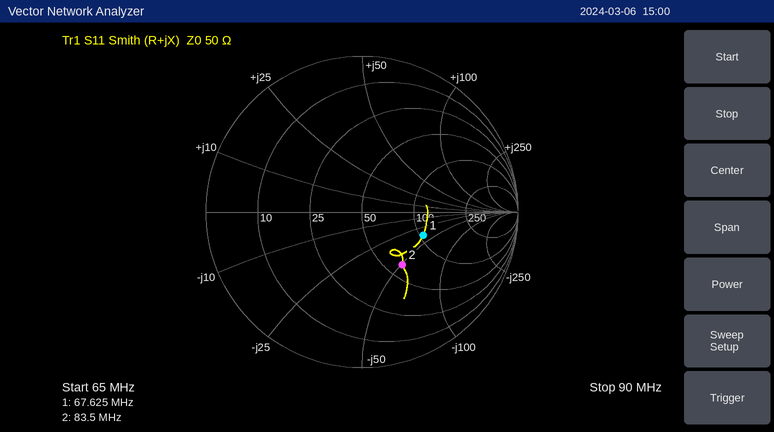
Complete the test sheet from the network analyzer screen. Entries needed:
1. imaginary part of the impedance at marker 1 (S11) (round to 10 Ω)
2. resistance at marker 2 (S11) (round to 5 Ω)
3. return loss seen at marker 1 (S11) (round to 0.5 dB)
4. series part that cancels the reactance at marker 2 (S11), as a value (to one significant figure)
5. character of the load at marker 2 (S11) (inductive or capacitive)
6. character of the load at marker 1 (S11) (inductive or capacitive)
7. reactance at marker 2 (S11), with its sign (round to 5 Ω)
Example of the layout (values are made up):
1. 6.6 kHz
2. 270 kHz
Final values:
1. -40 Ω
2. 60 Ω
3. 7.5 dB
4. 100 nH
5. capacitive
6. capacitive
7. -50 Ω
